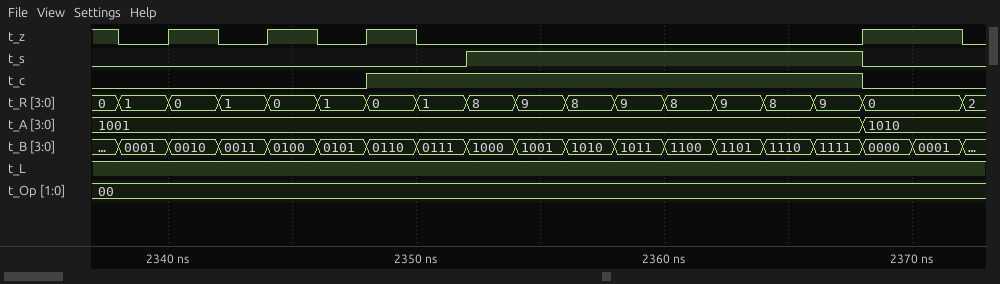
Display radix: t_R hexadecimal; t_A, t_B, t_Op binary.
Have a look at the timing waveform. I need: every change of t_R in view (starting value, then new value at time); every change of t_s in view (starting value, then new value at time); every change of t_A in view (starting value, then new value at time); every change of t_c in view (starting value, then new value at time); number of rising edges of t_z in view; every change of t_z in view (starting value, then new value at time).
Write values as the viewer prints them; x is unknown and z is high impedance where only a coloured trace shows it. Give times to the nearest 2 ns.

0, 1 at 2338 ns, 0 at 2340 ns, 1 at 2342 ns, 0 at 2344 ns, 1 at 2346 ns, 0 at 2348 ns, 1 at 2350 ns, 8 at 2352 ns, 9 at 2354 ns, 8 at 2356 ns, 9 at 2358 ns, 8 at 2360 ns, 9 at 2362 ns, 8 at 2364 ns, 9 at 2366 ns, 0 at 2368 ns, 2 at 2372 ns
0, 1 at 2352 ns, 0 at 2368 ns
1001, 1010 at 2368 ns
0, 1 at 2348 ns, 0 at 2368 ns
4
1, 0 at 2338 ns, 1 at 2340 ns, 0 at 2342 ns, 1 at 2344 ns, 0 at 2346 ns, 1 at 2348 ns, 0 at 2350 ns, 1 at 2368 ns, 0 at 2372 ns
